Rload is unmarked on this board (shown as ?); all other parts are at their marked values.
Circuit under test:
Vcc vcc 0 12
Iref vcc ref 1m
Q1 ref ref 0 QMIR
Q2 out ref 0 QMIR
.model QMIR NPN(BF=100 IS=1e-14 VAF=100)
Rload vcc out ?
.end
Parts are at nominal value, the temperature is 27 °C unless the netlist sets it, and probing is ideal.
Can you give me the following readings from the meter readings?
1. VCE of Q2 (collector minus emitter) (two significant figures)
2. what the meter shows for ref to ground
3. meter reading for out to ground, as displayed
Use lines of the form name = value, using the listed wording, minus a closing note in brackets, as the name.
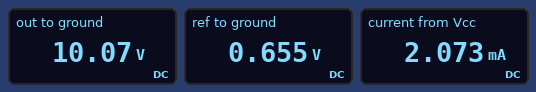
VCE of Q2 (collector minus emitter) = 10 V
what the meter shows for ref to ground = 0.655 V
meter reading for out to ground, as displayed = 10.07 V
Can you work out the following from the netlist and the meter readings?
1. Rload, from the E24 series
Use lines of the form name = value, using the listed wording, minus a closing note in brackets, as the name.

Rload, from the E24 series = 1.8 kΩ
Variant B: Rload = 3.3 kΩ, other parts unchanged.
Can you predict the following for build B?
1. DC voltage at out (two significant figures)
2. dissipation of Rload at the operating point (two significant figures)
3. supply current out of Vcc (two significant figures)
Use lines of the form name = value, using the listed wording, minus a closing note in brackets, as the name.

DC voltage at out = 8.5 V
dissipation of Rload at the operating point = 3.7 mW
supply current out of Vcc = 2.1 mA
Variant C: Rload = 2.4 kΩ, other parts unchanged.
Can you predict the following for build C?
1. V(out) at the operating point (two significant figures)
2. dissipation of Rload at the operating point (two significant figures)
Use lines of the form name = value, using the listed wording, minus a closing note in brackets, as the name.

V(out) at the operating point = 9.4 V
dissipation of Rload at the operating point = 2.7 mW
